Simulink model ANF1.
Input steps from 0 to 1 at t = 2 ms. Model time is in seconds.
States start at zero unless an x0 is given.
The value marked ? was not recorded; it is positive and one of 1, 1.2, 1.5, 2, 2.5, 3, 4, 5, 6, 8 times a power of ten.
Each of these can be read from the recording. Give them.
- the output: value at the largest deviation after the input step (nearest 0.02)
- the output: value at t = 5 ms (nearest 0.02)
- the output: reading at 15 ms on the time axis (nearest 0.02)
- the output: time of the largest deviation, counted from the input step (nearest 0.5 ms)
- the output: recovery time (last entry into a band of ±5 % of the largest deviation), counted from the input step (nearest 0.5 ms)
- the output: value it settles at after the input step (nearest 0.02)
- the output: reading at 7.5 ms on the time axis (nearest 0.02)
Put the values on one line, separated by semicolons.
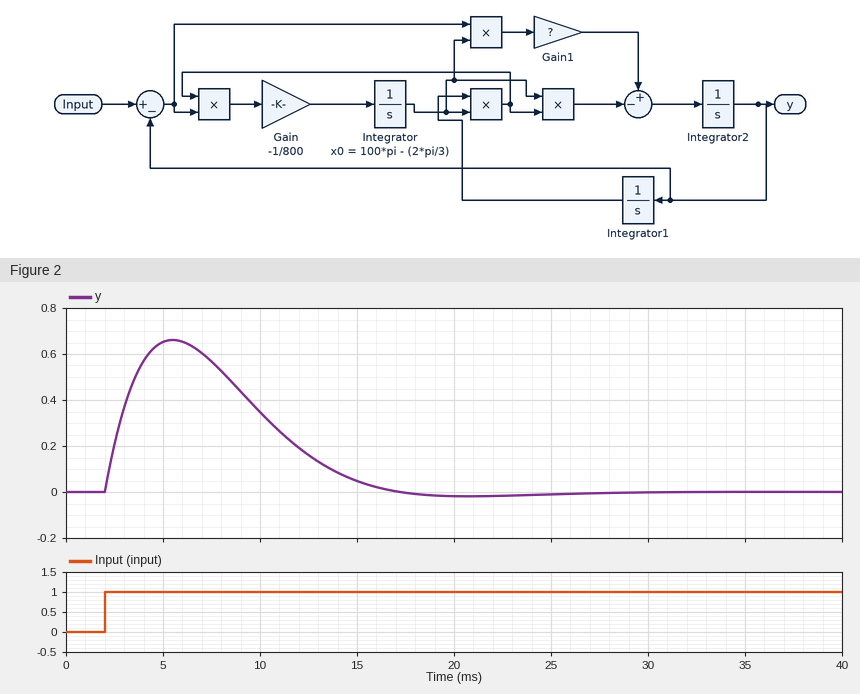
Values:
0.66; 0.66; 0.04; 3.5 ms; 13.5 ms; 0.00; 0.56
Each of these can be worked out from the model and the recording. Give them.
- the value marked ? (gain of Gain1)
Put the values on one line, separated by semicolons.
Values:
1.5
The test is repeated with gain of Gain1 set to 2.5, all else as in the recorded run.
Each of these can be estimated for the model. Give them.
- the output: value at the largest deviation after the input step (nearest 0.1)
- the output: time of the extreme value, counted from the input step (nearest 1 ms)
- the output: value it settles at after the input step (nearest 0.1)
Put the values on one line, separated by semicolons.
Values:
0.8; 3 ms; 0.0
